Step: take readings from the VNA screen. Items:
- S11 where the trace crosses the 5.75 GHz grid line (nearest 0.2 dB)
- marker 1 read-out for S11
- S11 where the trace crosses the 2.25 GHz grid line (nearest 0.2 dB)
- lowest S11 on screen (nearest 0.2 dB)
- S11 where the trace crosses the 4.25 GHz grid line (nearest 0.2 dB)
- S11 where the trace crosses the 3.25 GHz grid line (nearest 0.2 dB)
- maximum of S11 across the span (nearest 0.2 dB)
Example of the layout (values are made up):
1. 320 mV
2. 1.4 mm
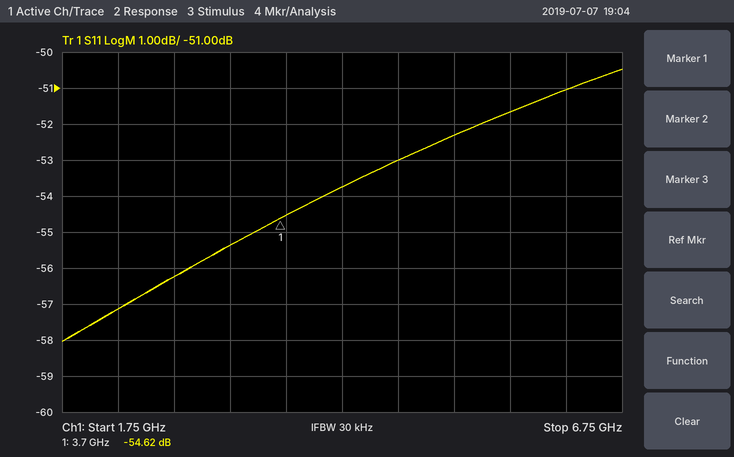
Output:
1. -51.6 dB
2. -54.62 dB
3. -57.2 dB
4. -58.0 dB
5. -53.8 dB
6. -55.4 dB
7. -50.4 dB
